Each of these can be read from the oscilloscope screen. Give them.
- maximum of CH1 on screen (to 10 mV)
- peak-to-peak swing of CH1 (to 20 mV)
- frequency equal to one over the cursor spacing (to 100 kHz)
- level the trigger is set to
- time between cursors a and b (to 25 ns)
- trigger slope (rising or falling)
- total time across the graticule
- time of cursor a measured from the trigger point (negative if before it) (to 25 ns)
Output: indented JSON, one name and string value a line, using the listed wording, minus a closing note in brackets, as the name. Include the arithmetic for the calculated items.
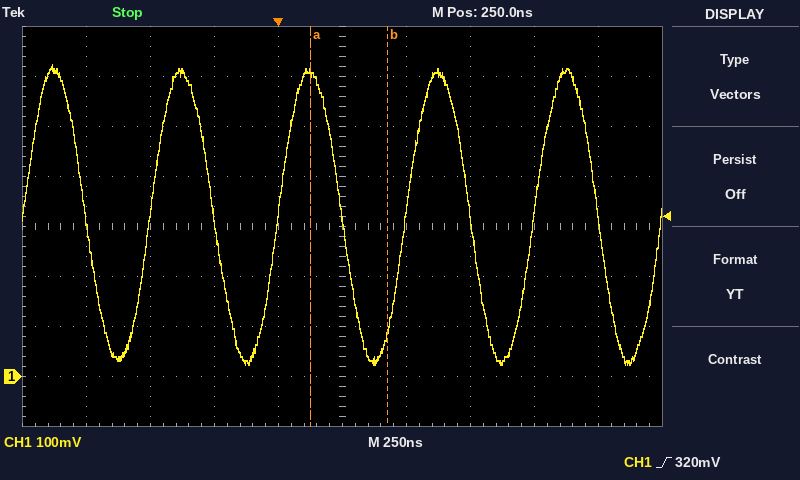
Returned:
{
  "maximum of CH1 on screen": "620 mV",
  "peak-to-peak swing of CH1": "600 mV",
  "frequency equal to one over the cursor spacing": "1 / 300 ns ≈ 3.3 MHz",
  "level the trigger is set to": "320 mV",
  "time between cursors a and b": "300 ns",
  "trigger slope": "rising",
  "total time across the graticule": "2.5 µs",
  "time of cursor a measured from the trigger point (negative if before it)": "+125 ns"
}
